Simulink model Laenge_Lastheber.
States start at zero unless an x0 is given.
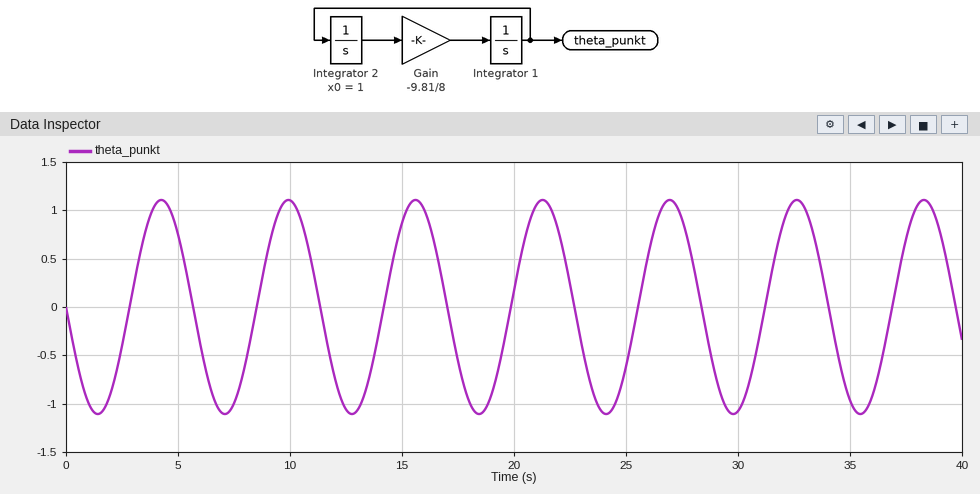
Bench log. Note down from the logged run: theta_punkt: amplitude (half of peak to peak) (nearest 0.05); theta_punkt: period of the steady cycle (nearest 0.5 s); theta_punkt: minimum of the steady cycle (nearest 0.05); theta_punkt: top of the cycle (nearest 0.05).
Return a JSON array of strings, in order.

["1.10", "5.5 s", "-1.10", "1.10"]
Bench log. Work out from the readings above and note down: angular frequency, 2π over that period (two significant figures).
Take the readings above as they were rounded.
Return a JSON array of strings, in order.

["1.1 rad/s"]
